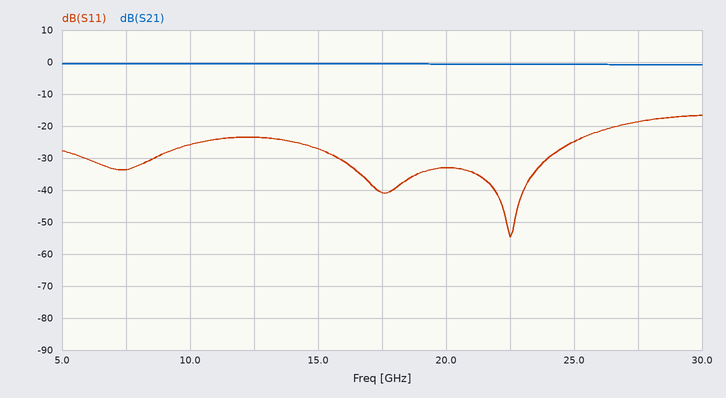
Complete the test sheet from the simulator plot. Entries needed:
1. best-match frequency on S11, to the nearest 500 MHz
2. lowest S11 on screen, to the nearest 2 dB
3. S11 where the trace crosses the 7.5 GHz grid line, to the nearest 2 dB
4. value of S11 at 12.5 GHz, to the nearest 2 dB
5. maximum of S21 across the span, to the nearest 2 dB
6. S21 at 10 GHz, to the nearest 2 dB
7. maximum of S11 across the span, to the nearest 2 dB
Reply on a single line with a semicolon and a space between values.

22.5 GHz; -54 dB; -34 dB; -24 dB; 0 dB; 0 dB; -16 dB
